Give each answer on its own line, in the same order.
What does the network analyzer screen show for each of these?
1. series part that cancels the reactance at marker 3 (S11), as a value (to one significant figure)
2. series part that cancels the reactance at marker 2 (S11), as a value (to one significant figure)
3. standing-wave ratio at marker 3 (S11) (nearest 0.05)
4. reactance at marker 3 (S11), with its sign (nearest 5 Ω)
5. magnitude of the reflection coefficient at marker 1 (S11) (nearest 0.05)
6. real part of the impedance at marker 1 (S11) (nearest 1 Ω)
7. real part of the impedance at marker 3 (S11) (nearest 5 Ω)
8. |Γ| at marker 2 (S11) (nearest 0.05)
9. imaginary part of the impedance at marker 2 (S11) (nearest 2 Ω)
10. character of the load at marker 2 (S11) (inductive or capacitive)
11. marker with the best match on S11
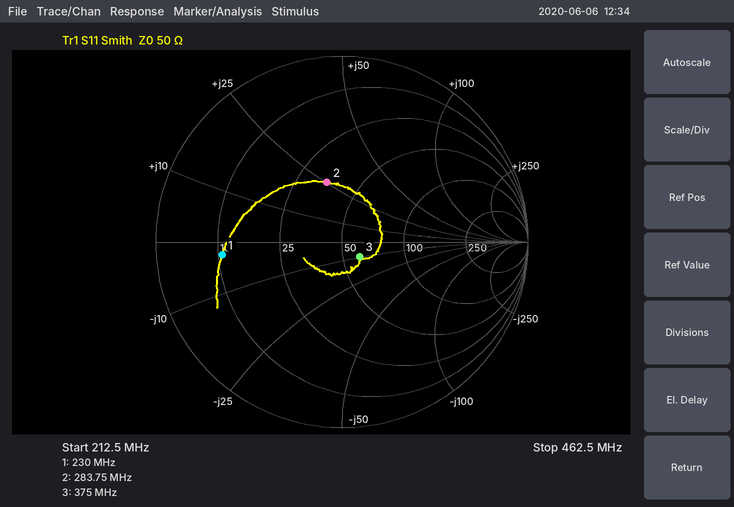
4 nH
20 pF
1.30
-10 Ω
0.65
11 Ω
60 Ω
0.35
+26 Ω
inductive
marker 3
